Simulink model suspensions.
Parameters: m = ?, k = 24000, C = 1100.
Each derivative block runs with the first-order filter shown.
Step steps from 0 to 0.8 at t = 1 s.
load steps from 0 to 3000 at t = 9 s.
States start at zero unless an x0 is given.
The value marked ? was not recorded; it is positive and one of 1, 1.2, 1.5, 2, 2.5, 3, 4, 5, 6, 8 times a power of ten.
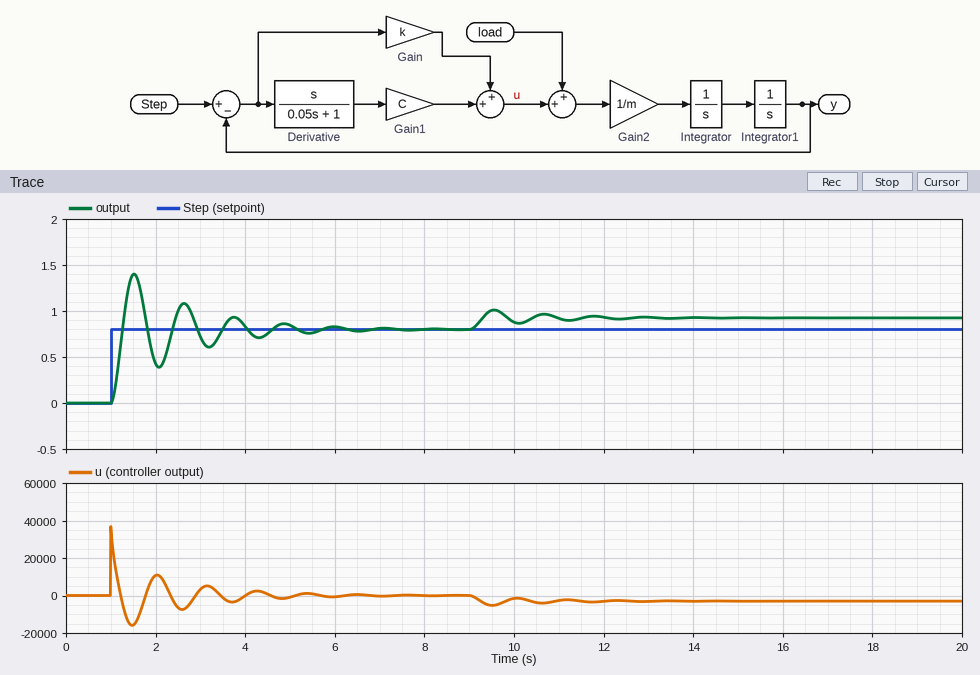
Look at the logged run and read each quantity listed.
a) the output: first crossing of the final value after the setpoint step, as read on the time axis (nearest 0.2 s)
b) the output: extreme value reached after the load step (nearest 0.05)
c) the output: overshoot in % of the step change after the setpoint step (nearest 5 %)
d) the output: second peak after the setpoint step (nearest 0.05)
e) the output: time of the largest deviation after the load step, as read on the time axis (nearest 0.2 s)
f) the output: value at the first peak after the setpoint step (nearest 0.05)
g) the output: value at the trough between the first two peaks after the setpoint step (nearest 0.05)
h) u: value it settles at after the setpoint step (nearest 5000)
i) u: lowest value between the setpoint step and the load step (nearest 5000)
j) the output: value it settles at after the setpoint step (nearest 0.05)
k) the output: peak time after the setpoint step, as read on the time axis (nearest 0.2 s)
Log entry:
1.2 s
1.00
75 %
1.10
9.6 s
1.40
0.40
0
-15000
0.80
1.6 s
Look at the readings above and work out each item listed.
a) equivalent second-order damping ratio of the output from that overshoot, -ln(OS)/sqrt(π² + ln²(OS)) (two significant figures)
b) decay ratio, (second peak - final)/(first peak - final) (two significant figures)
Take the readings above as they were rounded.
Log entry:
0.091
0.50
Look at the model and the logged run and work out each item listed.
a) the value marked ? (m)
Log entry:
800
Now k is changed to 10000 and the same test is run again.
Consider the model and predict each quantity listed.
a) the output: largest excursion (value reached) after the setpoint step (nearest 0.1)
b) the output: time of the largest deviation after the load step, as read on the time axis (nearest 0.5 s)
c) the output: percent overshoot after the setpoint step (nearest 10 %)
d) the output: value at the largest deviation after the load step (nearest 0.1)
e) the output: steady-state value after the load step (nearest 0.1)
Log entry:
1.3
10.0 s
60 %
1.3
1.1
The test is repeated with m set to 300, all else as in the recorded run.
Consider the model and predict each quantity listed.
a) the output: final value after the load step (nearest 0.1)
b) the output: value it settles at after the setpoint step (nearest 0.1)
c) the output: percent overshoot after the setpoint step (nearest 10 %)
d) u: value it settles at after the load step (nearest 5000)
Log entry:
0.9
0.8
70 %
-5000
